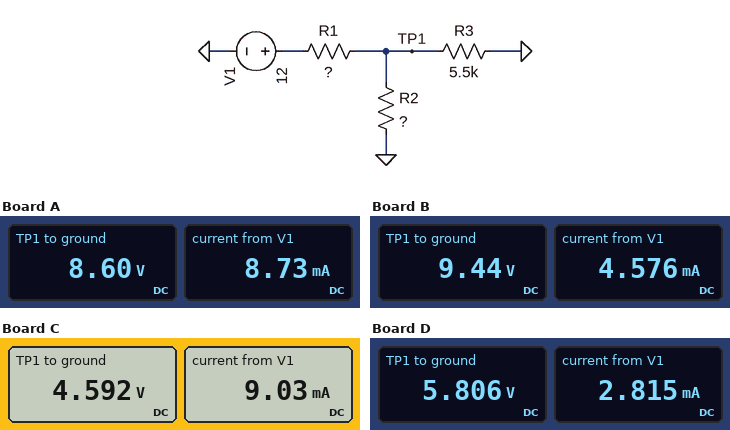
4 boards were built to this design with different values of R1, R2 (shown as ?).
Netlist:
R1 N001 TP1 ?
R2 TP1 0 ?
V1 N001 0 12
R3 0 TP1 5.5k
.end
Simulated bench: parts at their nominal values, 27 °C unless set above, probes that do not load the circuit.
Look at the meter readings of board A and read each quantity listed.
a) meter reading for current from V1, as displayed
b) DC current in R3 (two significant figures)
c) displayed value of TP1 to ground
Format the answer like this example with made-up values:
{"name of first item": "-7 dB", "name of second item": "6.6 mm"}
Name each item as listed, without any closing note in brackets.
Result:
{"meter reading for current from V1, as displayed": "8.73 mA", "DC current in R3": "1.6 mA", "displayed value of TP1 to ground": "8.60 V"}
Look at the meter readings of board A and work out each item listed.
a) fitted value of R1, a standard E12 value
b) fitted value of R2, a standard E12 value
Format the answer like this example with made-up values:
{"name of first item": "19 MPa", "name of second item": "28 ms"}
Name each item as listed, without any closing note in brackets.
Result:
{"fitted value of R1, a standard E12 value": "390 Ω", "fitted value of R2, a standard E12 value": "1.2 kΩ"}
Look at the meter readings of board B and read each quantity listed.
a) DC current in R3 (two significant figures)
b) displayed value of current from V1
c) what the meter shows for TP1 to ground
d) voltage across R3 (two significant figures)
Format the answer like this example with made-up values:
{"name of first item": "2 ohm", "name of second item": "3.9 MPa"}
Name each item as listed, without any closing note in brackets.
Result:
{"DC current in R3": "1.7 mA", "displayed value of current from V1": "4.576 mA", "what the meter shows for TP1 to ground": "9.44 V", "voltage across R3": "9.4 V"}
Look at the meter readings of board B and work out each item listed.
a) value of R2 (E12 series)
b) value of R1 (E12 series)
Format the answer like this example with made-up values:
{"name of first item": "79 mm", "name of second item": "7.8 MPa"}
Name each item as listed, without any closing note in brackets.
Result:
{"value of R2": "3.3 kΩ", "value of R1": "560 Ω"}
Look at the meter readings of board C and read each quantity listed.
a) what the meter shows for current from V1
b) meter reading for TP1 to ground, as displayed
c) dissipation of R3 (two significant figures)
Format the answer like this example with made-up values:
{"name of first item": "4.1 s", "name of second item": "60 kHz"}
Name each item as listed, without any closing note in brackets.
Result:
{"what the meter shows for current from V1": "9.03 mA", "meter reading for TP1 to ground, as displayed": "4.592 V", "dissipation of R3": "3.8 mW"}
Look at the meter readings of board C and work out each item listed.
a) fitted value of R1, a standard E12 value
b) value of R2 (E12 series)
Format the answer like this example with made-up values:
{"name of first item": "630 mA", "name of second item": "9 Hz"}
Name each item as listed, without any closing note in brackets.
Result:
{"fitted value of R1, a standard E12 value": "820 Ω", "value of R2": "560 Ω"}
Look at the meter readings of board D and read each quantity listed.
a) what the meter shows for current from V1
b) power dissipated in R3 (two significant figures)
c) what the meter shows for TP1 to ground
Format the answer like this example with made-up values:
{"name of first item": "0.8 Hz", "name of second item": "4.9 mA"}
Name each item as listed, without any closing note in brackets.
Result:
{"what the meter shows for current from V1": "2.815 mA", "power dissipated in R3": "6.1 mW", "what the meter shows for TP1 to ground": "5.806 V"}
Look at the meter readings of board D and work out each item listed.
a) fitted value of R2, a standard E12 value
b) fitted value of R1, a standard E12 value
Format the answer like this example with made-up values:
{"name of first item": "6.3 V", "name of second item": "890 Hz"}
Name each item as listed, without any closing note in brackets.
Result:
{"fitted value of R2, a standard E12 value": "3.3 kΩ", "fitted value of R1, a standard E12 value": "2.2 kΩ"}
